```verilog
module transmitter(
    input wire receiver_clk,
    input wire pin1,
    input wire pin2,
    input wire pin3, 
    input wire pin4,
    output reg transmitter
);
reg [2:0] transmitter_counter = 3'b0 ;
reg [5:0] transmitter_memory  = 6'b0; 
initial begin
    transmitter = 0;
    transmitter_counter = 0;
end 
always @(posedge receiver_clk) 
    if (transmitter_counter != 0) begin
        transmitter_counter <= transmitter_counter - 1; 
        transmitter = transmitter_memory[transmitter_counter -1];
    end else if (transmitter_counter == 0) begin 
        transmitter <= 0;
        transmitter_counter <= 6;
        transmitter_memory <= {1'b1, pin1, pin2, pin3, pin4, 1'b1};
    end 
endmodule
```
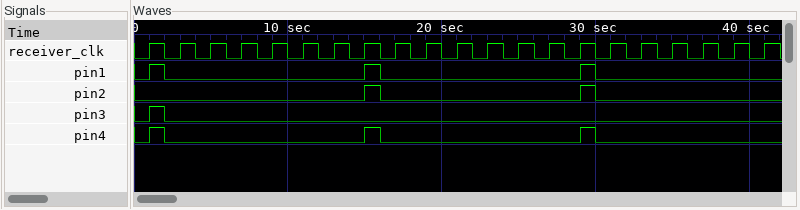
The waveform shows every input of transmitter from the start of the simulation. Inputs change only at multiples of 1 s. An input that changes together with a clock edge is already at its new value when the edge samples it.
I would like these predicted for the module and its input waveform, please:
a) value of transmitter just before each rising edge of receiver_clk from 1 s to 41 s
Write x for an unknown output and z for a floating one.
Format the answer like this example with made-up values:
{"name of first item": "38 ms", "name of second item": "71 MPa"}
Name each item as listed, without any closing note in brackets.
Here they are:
{"value of transmitter just before each rising edge of receiver_clk from 1 s to 41 s": "0 0 1 1 0 1 1 1 0 1 1 1 0 1 1 0 1 1 1 0 1"}
